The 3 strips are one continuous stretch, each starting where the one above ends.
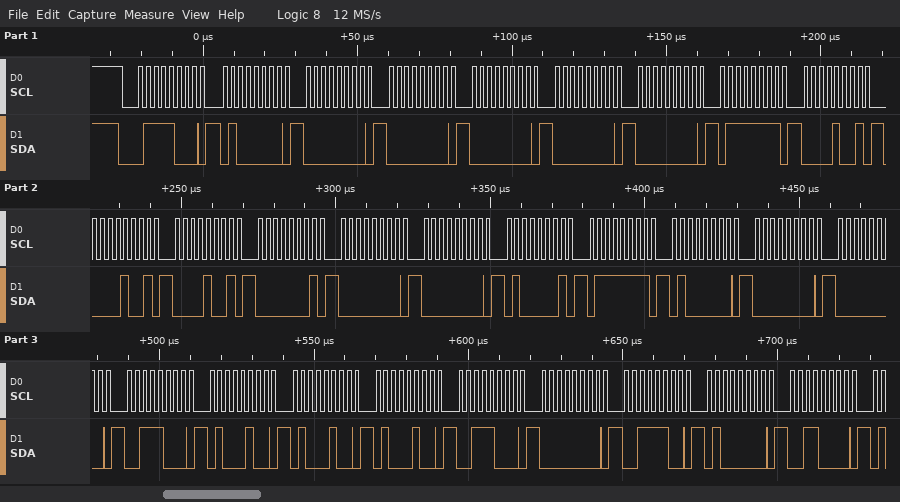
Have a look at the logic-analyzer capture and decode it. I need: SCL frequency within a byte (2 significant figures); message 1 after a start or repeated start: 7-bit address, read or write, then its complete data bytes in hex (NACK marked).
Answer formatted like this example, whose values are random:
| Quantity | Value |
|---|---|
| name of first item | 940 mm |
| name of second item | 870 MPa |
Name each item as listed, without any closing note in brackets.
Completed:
| Quantity | Value |
|---|---|
| SCL frequency within a byte | 400 kHz |
| message 1 after a start or repeated start: 7-bit address, read or write, then its complete data bytes in hex | 0x3C write: 40 00 00 00 00 00 7F 09 09 09 01 00 00 41 7F 40 00 00 38 44 44 44 38 00 3C 40 30 |
